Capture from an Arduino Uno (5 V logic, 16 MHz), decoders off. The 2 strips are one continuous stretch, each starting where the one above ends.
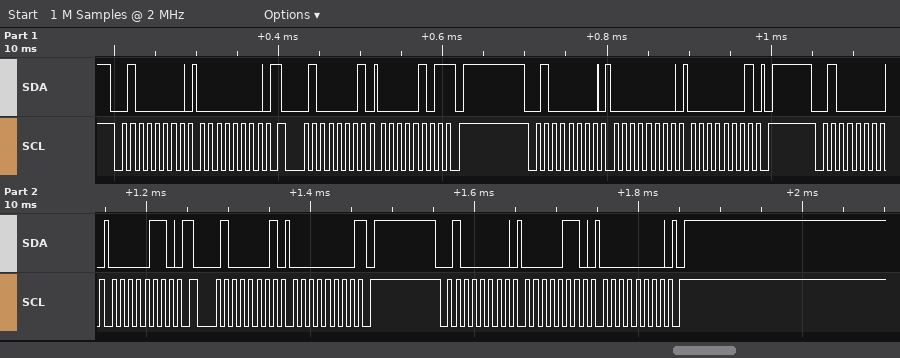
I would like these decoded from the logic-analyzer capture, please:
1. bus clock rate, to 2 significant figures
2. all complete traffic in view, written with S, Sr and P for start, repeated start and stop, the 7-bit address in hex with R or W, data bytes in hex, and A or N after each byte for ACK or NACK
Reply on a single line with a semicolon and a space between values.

100 kHz; S 20W A 00 A Sr 20R A 05 N P S 20W A 00 A 01 A P S 20W A 06 A Sr 20R A 00 N P S 20W A 06 A 00 A P
